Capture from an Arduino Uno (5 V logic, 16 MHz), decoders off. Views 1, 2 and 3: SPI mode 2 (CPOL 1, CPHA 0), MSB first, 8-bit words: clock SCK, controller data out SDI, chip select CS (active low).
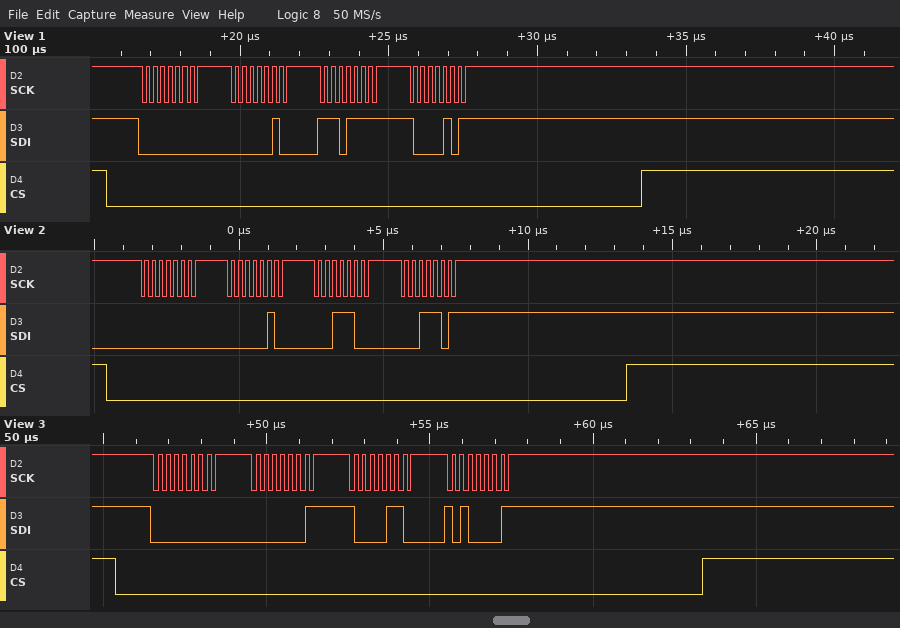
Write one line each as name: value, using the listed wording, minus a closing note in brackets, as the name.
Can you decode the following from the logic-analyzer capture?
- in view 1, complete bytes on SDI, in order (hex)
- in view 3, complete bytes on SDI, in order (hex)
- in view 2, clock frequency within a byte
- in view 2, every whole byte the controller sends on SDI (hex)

in view 1, complete bytes on SDI, in order: 00 02 EF 85
in view 3, complete bytes on SDI, in order: 00 01 86 A1
in view 2, clock frequency within a byte: 4 MHz
in view 2, every whole byte the controller sends on SDI: 00 02 1C 1D
